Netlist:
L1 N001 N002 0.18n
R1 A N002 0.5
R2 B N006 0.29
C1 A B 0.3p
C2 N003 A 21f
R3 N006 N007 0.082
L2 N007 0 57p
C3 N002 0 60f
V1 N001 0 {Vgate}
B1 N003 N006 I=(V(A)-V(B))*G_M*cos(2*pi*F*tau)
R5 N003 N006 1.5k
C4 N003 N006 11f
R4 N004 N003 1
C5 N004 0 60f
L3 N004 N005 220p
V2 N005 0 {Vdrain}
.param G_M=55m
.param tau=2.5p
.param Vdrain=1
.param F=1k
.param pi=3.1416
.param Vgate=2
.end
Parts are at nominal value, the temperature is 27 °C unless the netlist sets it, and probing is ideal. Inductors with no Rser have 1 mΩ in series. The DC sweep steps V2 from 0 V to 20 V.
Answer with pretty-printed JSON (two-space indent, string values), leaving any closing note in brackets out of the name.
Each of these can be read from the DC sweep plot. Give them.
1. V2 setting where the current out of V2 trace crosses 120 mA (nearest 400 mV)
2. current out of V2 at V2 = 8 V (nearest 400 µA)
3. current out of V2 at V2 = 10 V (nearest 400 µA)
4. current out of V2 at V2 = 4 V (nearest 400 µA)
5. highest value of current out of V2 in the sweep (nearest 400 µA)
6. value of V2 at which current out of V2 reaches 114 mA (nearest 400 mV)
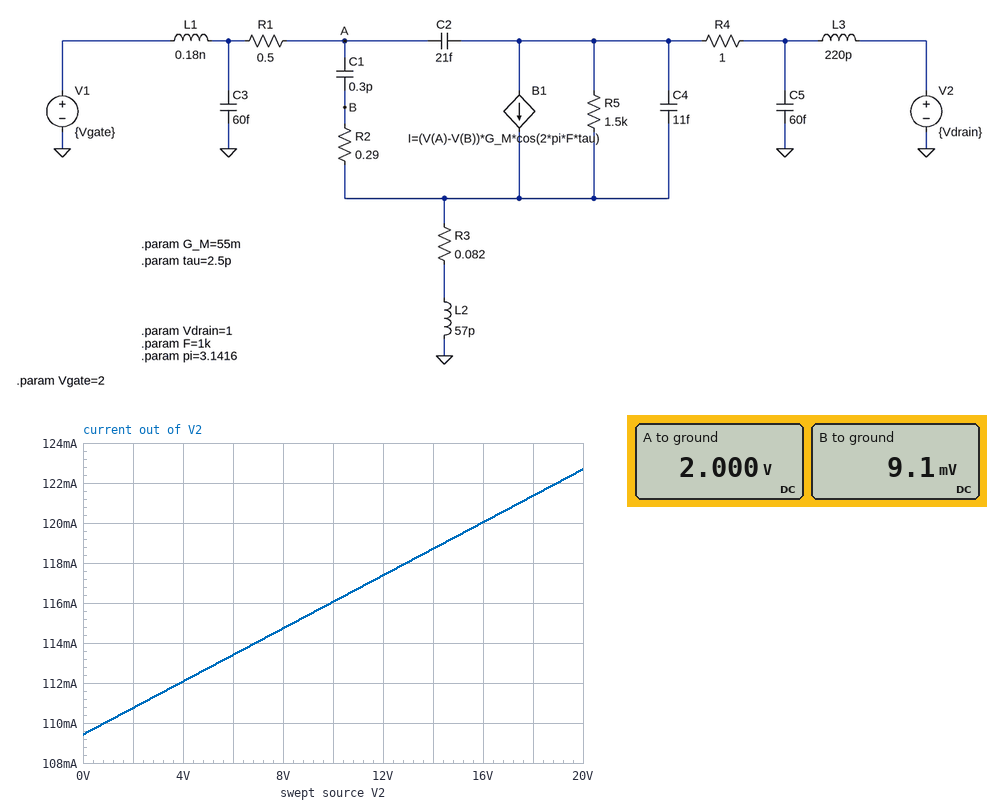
{
  "V2 setting where the current out of V2 trace crosses 120 mA": "16.0 V",
  "current out of V2 at V2 = 8 V": "114.8 mA",
  "current out of V2 at V2 = 10 V": "116.0 mA",
  "current out of V2 at V2 = 4 V": "112.0 mA",
  "highest value of current out of V2 in the sweep": "122.8 mA",
  "value of V2 at which current out of V2 reaches 114 mA": "6.8 V"
}
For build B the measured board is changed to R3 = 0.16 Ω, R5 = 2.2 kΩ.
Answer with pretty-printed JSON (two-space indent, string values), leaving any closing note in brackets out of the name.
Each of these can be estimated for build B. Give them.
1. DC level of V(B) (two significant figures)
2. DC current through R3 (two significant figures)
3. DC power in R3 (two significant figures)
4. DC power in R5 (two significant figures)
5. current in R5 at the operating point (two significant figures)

{
  "DC level of V(B)": "18 mV",
  "DC current through R3": "110 mA",
  "DC power in R3": "1.9 mW",
  "DC power in R5": "350 µW",
  "current in R5 at the operating point": "400 µA"
}
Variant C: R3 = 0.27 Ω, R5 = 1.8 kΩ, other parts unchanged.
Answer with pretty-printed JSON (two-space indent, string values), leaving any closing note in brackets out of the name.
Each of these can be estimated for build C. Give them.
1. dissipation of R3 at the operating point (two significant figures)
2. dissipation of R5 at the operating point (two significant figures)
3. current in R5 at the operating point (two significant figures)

{
  "dissipation of R3 at the operating point": "3.2 mW",
  "dissipation of R5 at the operating point": "410 µW",
  "current in R5 at the operating point": "480 µA"
}
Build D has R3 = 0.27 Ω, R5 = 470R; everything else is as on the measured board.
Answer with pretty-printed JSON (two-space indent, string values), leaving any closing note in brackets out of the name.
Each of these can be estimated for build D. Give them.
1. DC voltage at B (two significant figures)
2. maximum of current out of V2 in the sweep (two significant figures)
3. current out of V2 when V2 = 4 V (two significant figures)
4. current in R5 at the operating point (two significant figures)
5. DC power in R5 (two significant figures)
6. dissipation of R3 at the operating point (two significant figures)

{
  "DC voltage at B": "30 mV",
  "maximum of current out of V2 in the sweep": "150 mA",
  "current out of V2 when V2 = 4 V": "120 mA",
  "current in R5 at the operating point": "1.8 mA",
  "DC power in R5": "1.6 mW",
  "dissipation of R3 at the operating point": "3.3 mW"
}
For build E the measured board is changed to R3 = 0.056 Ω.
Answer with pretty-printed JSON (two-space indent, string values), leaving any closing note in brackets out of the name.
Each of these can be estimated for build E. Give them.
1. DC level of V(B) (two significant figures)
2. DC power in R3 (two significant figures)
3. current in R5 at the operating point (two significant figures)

{
  "DC level of V(B)": "6.3 mV",
  "DC power in R3": "680 µW",
  "current in R5 at the operating point": "590 µA"
}
